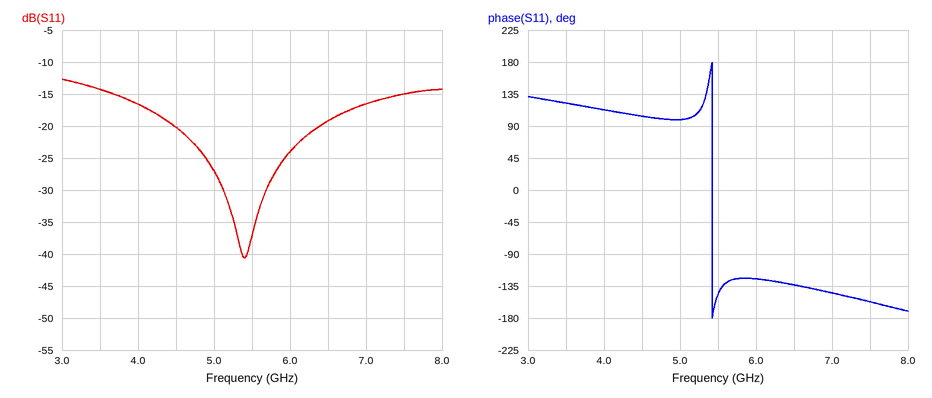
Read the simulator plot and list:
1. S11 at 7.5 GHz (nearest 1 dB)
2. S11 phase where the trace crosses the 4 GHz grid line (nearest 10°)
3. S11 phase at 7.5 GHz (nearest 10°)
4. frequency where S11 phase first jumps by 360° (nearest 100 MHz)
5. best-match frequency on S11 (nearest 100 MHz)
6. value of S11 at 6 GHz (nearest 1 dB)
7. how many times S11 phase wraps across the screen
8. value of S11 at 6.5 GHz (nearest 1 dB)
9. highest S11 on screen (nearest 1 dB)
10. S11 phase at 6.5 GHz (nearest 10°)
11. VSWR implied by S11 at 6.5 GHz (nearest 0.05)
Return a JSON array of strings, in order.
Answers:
["-15 dB", "110°", "-160°", "5.4 GHz", "5.4 GHz", "-24 dB", "1", "-19 dB", "-13 dB", "-130°", "1.25"]
